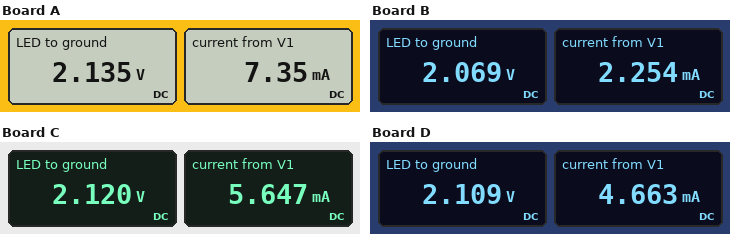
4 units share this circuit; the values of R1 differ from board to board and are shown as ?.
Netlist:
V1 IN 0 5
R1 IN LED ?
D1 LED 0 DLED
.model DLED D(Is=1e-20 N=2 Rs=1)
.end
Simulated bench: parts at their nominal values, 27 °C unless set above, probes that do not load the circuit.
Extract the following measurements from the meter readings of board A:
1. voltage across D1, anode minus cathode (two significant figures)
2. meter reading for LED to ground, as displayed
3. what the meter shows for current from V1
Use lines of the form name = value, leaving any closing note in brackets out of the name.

voltage across D1, anode minus cathode = 2.1 V
meter reading for LED to ground, as displayed = 2.135 V
what the meter shows for current from V1 = 7.35 mA
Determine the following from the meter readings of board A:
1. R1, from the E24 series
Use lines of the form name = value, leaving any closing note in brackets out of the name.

R1, from the E24 series = 390 Ω
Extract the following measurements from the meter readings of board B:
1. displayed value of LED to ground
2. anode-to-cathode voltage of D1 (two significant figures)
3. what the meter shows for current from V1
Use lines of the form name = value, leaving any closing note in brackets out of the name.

displayed value of LED to ground = 2.069 V
anode-to-cathode voltage of D1 = 2.1 V
what the meter shows for current from V1 = 2.254 mA
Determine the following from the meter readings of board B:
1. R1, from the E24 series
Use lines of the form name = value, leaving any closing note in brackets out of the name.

R1, from the E24 series = 1.3 kΩ
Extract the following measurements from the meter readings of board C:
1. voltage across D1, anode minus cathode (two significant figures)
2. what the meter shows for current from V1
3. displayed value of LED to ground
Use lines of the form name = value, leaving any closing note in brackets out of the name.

voltage across D1, anode minus cathode = 2.1 V
what the meter shows for current from V1 = 5.647 mA
displayed value of LED to ground = 2.120 V
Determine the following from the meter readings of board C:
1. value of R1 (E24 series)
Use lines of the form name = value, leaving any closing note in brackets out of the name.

value of R1 = 510 Ω
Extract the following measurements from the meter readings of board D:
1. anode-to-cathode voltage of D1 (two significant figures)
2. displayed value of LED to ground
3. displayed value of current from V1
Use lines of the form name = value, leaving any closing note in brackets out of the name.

anode-to-cathode voltage of D1 = 2.1 V
displayed value of LED to ground = 2.109 V
displayed value of current from V1 = 4.663 mA
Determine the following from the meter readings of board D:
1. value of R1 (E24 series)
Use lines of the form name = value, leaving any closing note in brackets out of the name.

value of R1 = 620 Ω
